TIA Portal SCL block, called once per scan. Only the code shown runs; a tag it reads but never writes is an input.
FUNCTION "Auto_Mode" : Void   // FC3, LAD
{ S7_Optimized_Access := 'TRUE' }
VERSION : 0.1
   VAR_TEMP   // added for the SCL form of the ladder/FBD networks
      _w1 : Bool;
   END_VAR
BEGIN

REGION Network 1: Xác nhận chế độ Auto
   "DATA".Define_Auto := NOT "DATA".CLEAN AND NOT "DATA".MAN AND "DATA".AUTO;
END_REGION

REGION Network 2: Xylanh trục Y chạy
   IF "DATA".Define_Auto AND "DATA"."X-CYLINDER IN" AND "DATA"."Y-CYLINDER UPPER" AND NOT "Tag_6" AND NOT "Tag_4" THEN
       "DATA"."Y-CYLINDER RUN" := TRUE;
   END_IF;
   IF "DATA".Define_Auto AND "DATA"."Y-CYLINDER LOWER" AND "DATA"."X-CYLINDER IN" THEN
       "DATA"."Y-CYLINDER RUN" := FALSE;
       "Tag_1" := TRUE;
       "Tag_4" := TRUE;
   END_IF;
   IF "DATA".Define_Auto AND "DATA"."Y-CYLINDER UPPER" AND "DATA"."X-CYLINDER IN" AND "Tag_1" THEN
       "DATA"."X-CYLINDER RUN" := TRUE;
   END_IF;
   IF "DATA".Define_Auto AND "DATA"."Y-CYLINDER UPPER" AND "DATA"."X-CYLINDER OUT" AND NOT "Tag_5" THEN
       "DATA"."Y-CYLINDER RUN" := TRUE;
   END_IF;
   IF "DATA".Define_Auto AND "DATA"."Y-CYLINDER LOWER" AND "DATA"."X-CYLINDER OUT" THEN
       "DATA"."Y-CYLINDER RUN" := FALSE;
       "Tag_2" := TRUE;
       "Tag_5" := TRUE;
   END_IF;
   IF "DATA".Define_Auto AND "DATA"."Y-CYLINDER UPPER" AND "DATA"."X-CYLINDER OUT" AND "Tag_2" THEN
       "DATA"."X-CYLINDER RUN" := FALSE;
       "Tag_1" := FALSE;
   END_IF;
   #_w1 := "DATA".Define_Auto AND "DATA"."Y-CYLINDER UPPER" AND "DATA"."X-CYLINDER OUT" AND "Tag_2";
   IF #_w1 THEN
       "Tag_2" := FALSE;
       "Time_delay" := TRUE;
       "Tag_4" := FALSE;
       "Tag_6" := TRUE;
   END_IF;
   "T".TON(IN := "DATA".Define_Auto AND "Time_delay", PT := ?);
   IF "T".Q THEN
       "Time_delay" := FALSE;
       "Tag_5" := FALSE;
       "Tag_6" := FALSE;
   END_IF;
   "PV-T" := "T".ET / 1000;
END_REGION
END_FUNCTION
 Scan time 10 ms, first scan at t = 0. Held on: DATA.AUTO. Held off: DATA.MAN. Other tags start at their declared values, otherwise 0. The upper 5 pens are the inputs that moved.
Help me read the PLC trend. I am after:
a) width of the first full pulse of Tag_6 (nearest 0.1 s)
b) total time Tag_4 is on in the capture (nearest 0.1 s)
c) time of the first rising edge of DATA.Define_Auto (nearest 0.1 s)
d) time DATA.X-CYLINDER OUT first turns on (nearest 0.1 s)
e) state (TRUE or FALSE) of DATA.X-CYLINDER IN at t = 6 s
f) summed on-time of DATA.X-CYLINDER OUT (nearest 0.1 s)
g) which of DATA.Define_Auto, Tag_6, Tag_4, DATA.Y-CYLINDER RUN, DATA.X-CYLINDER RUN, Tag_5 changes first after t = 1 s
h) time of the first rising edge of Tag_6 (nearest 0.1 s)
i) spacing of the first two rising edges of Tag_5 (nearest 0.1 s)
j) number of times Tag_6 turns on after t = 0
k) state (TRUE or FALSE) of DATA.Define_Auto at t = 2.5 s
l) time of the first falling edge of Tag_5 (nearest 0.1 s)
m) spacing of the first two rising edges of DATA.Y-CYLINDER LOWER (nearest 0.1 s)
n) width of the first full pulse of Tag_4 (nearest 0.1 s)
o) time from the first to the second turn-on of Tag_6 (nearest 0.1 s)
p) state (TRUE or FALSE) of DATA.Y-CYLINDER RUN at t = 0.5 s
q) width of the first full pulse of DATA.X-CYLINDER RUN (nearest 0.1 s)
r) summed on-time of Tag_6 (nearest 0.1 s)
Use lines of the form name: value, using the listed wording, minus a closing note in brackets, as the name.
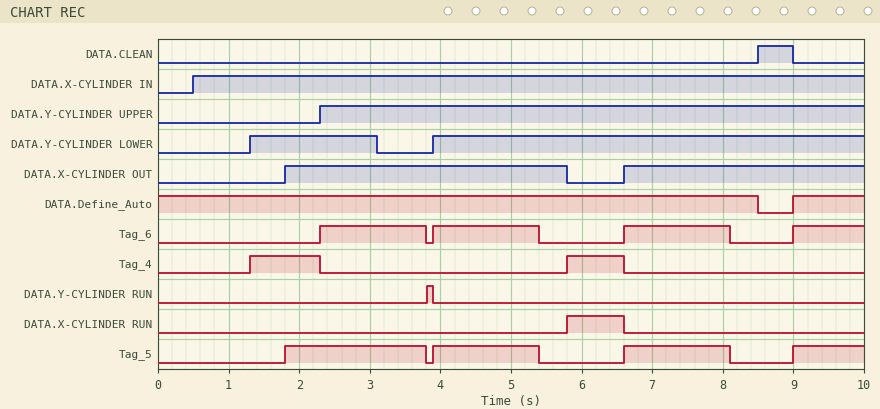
width of the first full pulse of Tag_6: 1.5 s
total time Tag_4 is on in the capture: 1.8 s
time of the first rising edge of DATA.Define_Auto: 9.0 s
time DATA.X-CYLINDER OUT first turns on: 1.8 s
state (TRUE or FALSE) of DATA.X-CYLINDER IN at t = 6 s: TRUE
summed on-time of DATA.X-CYLINDER OUT: 7.4 s
which of DATA.Define_Auto, Tag_6, Tag_4, DATA.Y-CYLINDER RUN, DATA.X-CYLINDER RUN, Tag_5 changes first after t = 1 s: Tag_4
time of the first rising edge of Tag_6: 2.3 s
spacing of the first two rising edges of Tag_5: 2.1 s
number of times Tag_6 turns on after t = 0: 4
state (TRUE or FALSE) of DATA.Define_Auto at t = 2.5 s: TRUE
time of the first falling edge of Tag_5: 3.8 s
spacing of the first two rising edges of DATA.Y-CYLINDER LOWER: 2.6 s
width of the first full pulse of Tag_4: 1.0 s
time from the first to the second turn-on of Tag_6: 1.6 s
state (TRUE or FALSE) of DATA.Y-CYLINDER RUN at t = 0.5 s: FALSE
width of the first full pulse of DATA.X-CYLINDER RUN: 0.8 s
summed on-time of Tag_6: 5.5 s
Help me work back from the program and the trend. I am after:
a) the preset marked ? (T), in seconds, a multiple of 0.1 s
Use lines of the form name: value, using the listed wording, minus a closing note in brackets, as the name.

the preset marked ? (T), in seconds, a multiple of 0.1 s: 1.5 s
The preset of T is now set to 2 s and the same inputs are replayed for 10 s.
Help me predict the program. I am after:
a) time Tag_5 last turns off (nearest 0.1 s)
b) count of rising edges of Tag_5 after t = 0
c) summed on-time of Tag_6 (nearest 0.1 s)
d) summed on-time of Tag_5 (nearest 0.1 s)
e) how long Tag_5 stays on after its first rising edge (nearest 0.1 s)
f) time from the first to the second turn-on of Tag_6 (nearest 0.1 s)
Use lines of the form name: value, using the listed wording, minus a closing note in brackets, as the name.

time Tag_5 last turns off: 4.3 s
count of rising edges of Tag_5 after t = 0: 2
summed on-time of Tag_6: 5.4 s
summed on-time of Tag_5: 5.9 s
how long Tag_5 stays on after its first rising edge: 2.5 s
time from the first to the second turn-on of Tag_6: 4.3 s
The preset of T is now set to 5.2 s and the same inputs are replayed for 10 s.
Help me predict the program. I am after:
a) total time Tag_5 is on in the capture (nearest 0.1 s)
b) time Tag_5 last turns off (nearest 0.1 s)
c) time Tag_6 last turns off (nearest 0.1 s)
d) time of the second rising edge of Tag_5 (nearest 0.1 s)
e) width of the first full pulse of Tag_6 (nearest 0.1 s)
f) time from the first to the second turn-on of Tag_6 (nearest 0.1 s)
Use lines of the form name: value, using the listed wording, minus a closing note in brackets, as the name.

total time Tag_5 is on in the capture: 6.7 s
time Tag_5 last turns off: 7.5 s
time Tag_6 last turns off: 7.5 s
time of the second rising edge of Tag_5: 9.0 s
width of the first full pulse of Tag_6: 5.2 s
time from the first to the second turn-on of Tag_6: 6.7 s
